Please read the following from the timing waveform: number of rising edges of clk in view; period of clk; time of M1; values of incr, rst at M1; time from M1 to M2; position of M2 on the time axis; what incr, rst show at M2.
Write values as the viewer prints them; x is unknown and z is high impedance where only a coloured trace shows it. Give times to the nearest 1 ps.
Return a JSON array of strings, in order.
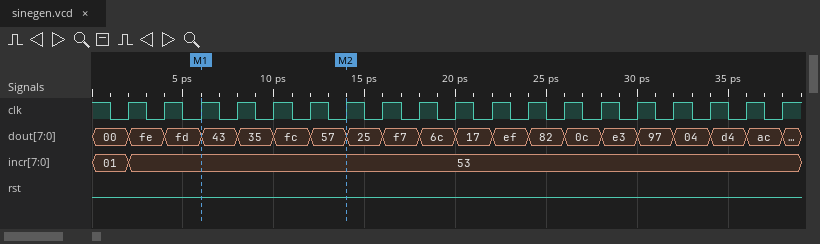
["19", "2 ps", "6 ps", "incr=53, rst=0", "8 ps", "14 ps", "incr=53, rst=0"]
